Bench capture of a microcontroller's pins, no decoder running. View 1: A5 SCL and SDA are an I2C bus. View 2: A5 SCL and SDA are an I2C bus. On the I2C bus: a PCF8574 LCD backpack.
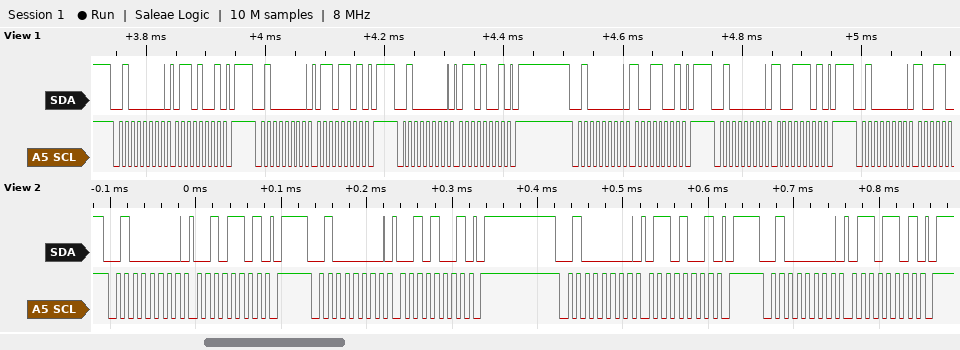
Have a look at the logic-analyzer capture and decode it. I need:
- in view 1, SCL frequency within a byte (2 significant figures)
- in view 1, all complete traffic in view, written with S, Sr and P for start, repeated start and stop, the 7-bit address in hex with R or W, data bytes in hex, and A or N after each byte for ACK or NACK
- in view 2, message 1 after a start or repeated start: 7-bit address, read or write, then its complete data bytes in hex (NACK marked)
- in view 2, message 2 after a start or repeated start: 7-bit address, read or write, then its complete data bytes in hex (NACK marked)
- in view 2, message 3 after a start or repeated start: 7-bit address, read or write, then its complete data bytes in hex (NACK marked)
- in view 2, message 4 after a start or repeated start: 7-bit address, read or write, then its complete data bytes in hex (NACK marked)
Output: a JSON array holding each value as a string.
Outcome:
["100 kHz", "S 20W A 69 A P S 20W A 6D A P S 20W A 69 A P S 20W A 99 A P S 20W A 9D A P S 20W A", "0x20 write: 2D", "0x20 write: 29", "0x20 write: 69", "0x20 write: 6D"]
